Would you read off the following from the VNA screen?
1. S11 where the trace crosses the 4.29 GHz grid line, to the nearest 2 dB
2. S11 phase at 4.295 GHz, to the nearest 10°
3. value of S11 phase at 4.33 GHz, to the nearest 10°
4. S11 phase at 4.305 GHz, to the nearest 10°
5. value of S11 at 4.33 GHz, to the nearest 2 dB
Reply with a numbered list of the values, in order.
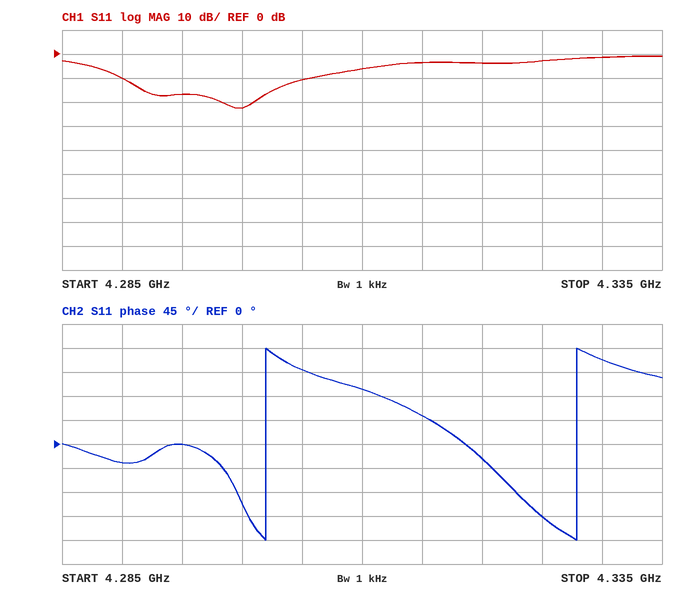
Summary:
1. -10 dB
2. 0°
3. 160°
4. 140°
5. -2 dB
